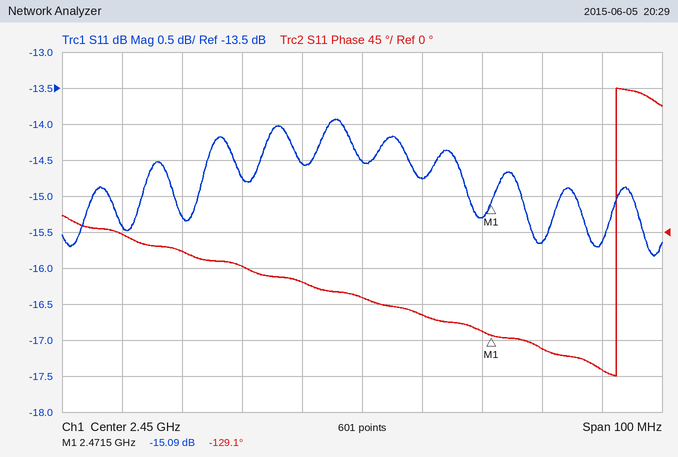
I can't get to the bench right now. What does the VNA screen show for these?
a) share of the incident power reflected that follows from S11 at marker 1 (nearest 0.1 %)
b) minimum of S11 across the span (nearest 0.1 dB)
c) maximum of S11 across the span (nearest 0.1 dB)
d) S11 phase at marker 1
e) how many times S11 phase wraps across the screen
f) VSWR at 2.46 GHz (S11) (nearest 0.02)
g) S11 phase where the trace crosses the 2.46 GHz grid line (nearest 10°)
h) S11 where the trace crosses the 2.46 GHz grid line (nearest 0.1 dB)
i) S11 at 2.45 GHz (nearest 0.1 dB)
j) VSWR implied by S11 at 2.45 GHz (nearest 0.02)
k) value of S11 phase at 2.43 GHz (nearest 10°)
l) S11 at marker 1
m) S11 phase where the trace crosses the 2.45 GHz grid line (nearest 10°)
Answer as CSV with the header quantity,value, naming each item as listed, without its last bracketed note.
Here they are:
quantity,value
share of the incident power reflected that follows from S11 at marker 1,3.1 %
minimum of S11 across the span,-15.8 dB
maximum of S11 across the span,-13.9 dB
S11 phase at marker 1,-129.1°
how many times S11 phase wraps across the screen,1
VSWR at 2.46 GHz (S11),1.44
S11 phase where the trace crosses the 2.46 GHz grid line,-100°
S11 where the trace crosses the 2.46 GHz grid line,-14.8 dB
S11 at 2.45 GHz,-14.5 dB
VSWR implied by S11 at 2.45 GHz,1.46
value of S11 phase at 2.43 GHz,-40°
S11 at marker 1,-15.09 dB
S11 phase where the trace crosses the 2.45 GHz grid line,-80°
